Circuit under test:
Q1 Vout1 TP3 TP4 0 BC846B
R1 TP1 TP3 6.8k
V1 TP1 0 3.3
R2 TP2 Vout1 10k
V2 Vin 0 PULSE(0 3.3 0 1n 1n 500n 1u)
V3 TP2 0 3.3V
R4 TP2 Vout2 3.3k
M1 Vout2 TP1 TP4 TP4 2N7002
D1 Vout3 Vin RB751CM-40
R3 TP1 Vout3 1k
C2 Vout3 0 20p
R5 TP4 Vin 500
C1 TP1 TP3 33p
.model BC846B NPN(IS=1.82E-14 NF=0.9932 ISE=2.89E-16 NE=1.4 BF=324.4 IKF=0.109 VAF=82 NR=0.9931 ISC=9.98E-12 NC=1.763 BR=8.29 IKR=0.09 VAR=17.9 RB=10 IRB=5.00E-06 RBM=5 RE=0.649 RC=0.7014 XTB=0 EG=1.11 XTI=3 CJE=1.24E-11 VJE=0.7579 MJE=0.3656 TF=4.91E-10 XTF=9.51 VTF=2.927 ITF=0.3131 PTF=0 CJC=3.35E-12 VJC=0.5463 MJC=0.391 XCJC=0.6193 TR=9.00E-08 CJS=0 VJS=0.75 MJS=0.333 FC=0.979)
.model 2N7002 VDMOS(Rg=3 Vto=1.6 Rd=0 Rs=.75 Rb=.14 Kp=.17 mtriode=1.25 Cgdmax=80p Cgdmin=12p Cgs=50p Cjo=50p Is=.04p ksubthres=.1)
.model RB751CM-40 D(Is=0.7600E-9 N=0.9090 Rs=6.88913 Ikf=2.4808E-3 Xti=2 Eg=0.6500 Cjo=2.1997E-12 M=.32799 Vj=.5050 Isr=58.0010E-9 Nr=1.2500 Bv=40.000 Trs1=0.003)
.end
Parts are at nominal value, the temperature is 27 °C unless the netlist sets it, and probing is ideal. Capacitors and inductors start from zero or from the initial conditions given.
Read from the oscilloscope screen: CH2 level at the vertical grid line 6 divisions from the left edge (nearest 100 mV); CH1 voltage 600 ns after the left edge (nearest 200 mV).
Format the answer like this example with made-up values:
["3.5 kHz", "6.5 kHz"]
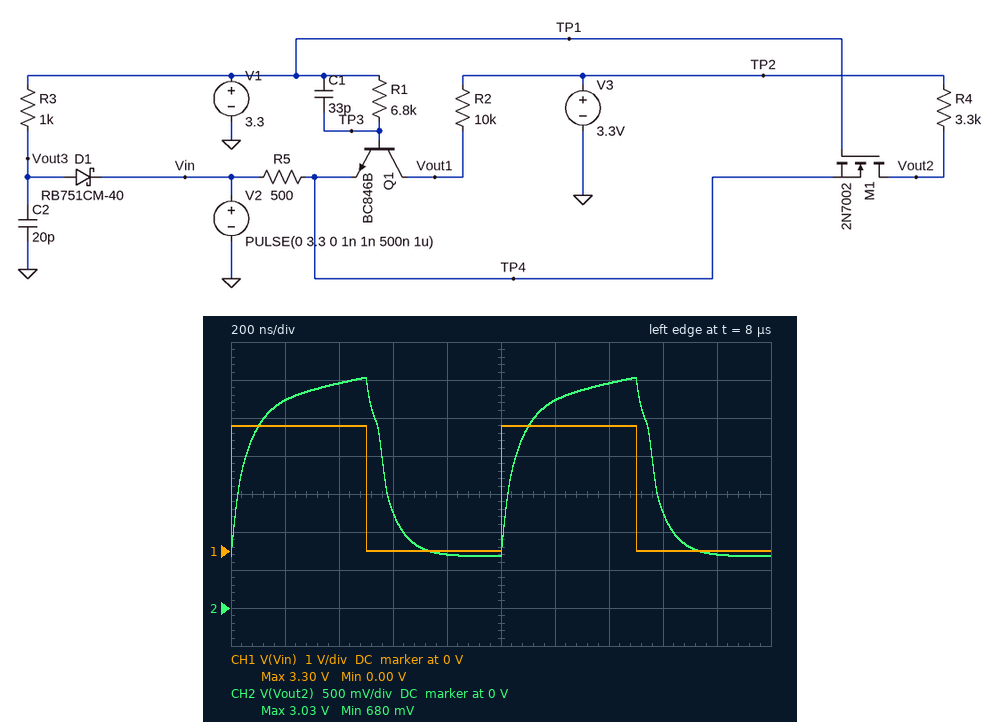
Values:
["2.7 V", "0 V"]
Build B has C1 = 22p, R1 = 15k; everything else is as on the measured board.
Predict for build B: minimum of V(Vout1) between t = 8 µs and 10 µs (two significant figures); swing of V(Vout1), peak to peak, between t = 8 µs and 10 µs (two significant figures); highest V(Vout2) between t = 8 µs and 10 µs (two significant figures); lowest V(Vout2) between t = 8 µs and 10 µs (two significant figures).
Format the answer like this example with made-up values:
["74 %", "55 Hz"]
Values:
["620 mV", "2.7 V", "3.0 V", "610 mV"]
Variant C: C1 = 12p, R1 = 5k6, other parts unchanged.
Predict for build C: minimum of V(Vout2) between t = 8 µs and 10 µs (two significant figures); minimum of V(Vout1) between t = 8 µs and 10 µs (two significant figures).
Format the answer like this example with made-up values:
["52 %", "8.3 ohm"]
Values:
["700 mV", "710 mV"]
